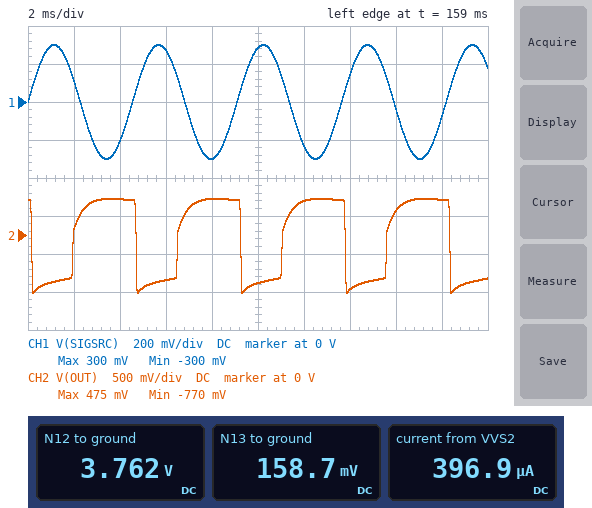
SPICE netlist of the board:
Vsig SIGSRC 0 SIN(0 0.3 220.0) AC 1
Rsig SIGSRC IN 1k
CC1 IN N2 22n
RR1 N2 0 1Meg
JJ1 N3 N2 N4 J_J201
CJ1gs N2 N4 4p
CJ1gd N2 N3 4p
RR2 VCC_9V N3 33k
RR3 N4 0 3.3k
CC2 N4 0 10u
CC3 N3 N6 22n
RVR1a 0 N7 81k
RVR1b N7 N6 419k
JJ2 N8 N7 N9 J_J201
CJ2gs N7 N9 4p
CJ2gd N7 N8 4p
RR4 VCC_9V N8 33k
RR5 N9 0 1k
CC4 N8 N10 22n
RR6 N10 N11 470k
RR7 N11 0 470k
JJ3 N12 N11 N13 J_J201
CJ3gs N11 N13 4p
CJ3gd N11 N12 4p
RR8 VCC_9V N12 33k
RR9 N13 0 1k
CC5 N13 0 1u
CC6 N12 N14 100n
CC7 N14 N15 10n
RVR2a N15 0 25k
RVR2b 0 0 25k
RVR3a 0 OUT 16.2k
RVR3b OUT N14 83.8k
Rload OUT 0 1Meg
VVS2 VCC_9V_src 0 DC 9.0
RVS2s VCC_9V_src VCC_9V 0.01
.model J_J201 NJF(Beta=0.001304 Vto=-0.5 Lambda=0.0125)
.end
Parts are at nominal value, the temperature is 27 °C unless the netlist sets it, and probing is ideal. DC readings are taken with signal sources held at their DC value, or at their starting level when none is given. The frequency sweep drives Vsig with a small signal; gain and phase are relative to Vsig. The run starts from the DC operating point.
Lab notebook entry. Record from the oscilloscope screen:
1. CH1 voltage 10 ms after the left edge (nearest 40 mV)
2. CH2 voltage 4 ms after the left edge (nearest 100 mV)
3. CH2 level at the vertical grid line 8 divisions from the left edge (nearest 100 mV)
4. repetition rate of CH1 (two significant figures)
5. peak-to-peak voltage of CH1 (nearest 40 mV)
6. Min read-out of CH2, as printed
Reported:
280 mV
500 mV
300 mV
220 Hz
600 mV
-770 mV
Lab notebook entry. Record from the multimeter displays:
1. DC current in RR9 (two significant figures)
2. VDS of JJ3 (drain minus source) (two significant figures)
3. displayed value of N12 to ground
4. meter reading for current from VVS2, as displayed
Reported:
160 µA
3.6 V
3.762 V
396.9 µA
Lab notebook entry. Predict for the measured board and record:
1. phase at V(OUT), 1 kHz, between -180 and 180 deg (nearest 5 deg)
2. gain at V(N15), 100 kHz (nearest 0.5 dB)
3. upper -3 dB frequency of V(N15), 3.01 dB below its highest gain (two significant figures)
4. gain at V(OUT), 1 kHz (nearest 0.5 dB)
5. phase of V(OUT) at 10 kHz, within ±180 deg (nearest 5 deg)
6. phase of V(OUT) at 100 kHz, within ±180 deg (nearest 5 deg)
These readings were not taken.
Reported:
170 deg
21.0 dB
12 kHz
33.5 dB
125 deg
20 deg
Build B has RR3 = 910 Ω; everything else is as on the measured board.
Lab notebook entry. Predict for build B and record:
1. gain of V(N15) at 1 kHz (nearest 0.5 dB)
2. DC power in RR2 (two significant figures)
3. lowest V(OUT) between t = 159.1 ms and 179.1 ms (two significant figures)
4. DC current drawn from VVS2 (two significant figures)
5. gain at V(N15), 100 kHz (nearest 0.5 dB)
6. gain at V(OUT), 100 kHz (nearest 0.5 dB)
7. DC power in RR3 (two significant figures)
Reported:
50.5 dB
910 µW
-650 mV
480 µA
23.5 dB
7.5 dB
25 µW
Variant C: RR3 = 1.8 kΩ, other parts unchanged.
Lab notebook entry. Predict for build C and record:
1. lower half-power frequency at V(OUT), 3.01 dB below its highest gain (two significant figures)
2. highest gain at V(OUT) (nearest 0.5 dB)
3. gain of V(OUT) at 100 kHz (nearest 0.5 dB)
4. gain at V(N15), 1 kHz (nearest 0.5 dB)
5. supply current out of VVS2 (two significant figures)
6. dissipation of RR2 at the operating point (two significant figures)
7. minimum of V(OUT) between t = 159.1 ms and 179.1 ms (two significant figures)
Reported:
50 Hz
36.0 dB
6.5 dB
49.5 dB
430 µA
450 µW
-710 mV
